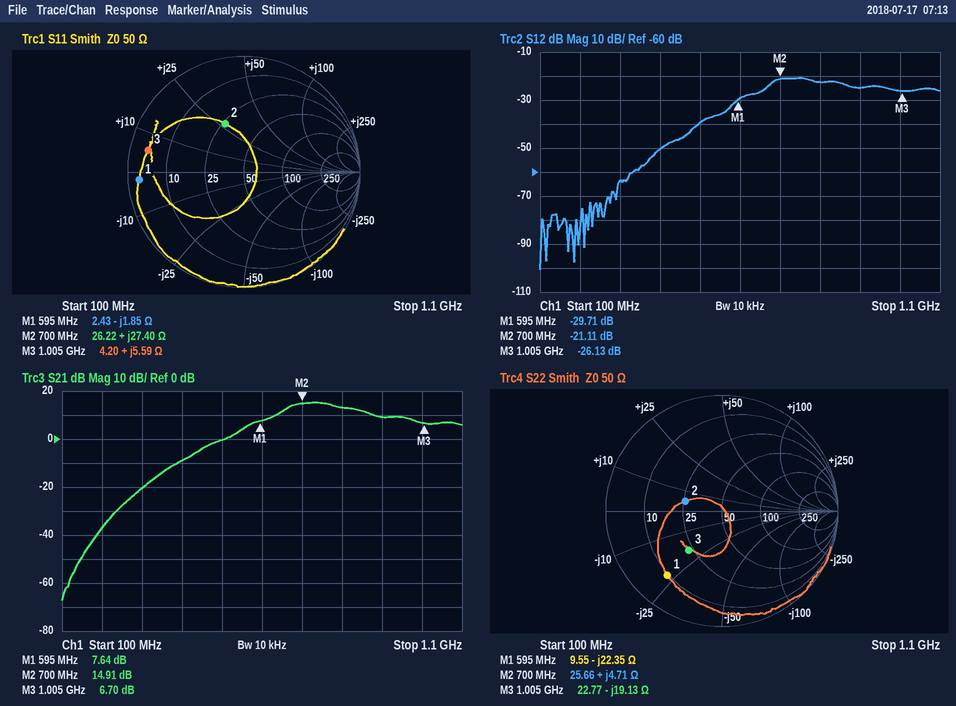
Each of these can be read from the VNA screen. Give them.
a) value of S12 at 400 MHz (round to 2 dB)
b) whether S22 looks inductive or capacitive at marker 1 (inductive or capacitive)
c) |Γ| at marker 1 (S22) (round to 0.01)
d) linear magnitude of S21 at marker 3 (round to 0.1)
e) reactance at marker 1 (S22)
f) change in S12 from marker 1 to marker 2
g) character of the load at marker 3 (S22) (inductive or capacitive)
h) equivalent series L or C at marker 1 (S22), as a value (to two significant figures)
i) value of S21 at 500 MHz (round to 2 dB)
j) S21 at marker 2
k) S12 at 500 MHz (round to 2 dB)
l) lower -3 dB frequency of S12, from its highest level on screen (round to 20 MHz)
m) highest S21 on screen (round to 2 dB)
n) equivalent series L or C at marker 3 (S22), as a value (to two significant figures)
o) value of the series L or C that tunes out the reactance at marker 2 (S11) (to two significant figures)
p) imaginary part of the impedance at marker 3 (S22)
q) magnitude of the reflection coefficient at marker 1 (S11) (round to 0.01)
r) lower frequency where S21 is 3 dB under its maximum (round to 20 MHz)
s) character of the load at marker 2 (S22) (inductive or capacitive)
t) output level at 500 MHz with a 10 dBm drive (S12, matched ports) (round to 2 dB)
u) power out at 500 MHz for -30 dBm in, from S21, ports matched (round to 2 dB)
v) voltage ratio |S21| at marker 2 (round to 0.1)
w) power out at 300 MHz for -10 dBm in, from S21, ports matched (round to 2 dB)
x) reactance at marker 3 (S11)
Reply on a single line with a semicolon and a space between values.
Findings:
-50 dB; capacitive; 0.73; 2.2; -22.35 Ω; 8.60 dB; capacitive; 12 pF; 0 dB; 14.91 dB; -40 dB; 680 MHz; 16 dB; 8.3 pF; 8.3 pF; -19.13 Ω; 0.91; 660 MHz; inductive; -30 dBm; -30 dBm; 5.6; -30 dBm; +5.59 Ω
